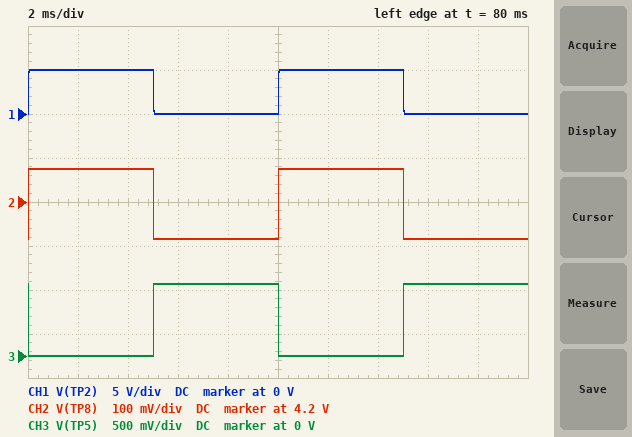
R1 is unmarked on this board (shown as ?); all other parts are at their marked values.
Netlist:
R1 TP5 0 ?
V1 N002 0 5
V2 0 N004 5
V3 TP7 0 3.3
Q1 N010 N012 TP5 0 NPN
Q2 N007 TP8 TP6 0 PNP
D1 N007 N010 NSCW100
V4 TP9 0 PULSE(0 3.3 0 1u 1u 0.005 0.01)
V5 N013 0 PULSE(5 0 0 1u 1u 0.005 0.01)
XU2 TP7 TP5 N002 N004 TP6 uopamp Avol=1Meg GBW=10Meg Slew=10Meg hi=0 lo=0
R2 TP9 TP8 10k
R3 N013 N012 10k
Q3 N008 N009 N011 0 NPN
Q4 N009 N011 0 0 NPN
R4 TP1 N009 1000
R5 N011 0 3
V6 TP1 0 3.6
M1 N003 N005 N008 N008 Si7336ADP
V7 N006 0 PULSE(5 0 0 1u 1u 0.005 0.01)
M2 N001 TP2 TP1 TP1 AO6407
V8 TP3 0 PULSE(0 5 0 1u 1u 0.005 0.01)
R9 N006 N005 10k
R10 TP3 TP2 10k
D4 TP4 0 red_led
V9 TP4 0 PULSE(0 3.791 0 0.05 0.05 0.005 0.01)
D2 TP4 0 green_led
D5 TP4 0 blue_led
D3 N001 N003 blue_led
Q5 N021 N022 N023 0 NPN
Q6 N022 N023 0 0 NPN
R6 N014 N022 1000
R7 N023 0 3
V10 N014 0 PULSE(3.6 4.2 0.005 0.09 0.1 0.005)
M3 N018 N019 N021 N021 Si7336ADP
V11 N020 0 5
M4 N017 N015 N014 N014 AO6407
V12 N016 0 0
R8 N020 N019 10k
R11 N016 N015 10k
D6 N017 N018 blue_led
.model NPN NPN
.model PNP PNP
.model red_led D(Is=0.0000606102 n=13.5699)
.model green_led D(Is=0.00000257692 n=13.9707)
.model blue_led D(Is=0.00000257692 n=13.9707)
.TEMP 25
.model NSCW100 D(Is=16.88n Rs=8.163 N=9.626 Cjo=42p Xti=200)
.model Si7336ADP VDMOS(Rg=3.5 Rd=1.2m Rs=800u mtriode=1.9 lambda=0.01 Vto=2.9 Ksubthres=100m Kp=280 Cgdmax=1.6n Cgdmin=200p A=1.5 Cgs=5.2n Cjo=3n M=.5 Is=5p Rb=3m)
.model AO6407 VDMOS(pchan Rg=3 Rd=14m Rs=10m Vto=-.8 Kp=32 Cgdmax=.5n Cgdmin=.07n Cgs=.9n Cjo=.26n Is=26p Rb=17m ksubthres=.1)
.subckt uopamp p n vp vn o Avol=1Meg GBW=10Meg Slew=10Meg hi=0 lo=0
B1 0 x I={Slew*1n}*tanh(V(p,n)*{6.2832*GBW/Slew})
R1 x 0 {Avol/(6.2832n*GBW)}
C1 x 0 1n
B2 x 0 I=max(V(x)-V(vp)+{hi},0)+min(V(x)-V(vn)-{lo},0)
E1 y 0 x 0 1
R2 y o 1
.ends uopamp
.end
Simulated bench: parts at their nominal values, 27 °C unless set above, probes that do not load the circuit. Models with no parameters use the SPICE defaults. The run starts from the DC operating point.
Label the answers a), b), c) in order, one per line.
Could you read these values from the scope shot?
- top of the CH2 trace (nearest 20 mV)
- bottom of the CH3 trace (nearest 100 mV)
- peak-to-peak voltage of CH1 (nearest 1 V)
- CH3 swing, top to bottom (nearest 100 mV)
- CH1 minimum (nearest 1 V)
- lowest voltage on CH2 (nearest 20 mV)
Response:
a) 4.28 V
b) 0 V
c) 5 V
d) 800 mV
e) 0 V
f) 4.12 V
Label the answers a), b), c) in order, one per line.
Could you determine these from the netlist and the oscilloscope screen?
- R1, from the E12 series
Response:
a) 27 Ω
